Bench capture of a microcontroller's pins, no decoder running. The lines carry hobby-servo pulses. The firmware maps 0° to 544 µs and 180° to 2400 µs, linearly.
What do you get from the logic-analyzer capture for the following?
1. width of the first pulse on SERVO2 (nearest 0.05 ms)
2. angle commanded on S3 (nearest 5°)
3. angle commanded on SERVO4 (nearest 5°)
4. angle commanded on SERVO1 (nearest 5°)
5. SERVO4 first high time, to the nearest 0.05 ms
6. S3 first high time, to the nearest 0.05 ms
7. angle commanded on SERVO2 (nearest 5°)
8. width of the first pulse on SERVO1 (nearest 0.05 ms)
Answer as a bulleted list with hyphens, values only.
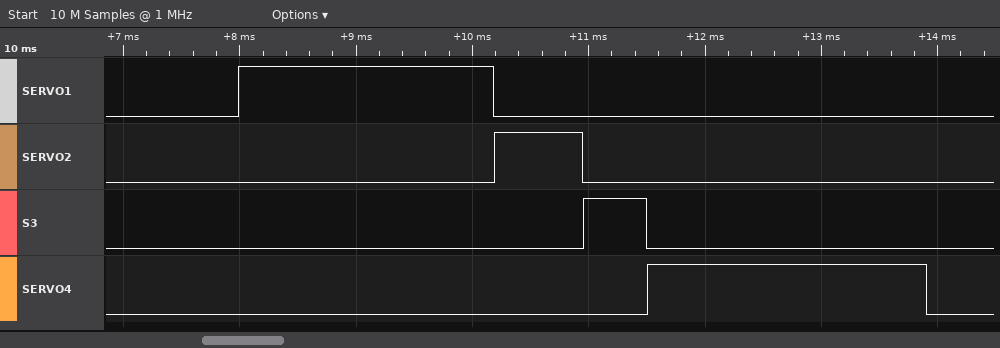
- 0.75 ms
- 0°
- 180°
- 160°
- 2.40 ms
- 0.55 ms
- 20°
- 2.20 ms
